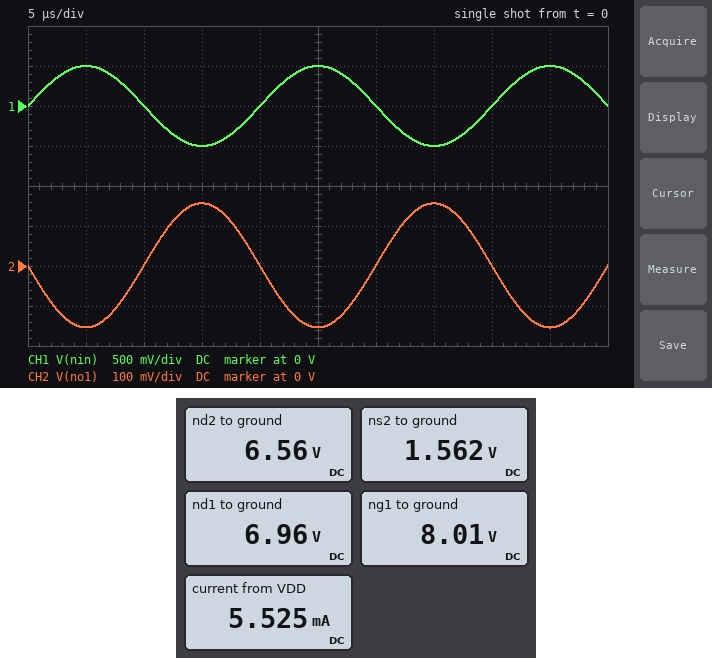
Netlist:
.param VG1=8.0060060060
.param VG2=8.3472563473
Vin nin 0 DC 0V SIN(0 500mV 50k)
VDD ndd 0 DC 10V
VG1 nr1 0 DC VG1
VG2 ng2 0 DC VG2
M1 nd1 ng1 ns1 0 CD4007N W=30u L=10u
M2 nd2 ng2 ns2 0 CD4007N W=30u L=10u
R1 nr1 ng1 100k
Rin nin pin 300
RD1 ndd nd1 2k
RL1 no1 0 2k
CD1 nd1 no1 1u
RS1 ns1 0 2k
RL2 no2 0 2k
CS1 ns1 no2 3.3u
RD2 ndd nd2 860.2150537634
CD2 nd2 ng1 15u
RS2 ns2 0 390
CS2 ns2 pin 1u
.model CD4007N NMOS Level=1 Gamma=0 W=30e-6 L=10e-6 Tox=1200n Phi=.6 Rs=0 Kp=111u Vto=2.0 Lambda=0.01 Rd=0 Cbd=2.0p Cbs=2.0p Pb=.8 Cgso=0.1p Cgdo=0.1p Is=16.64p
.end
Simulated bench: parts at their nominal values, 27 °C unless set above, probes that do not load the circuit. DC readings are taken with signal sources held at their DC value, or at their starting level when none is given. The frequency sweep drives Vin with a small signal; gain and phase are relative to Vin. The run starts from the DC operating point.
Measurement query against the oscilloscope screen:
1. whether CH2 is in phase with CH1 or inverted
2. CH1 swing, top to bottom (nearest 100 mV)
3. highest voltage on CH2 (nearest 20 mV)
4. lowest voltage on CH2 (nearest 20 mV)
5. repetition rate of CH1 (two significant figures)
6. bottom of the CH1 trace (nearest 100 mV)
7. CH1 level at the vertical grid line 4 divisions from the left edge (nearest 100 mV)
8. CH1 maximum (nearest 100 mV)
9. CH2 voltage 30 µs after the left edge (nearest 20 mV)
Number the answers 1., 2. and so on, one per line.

1. inverted
2. 1.0 V
3. 160 mV
4. -160 mV
5. 50 kHz
6. -500 mV
7. 0 V
8. 500 mV
9. 0 V
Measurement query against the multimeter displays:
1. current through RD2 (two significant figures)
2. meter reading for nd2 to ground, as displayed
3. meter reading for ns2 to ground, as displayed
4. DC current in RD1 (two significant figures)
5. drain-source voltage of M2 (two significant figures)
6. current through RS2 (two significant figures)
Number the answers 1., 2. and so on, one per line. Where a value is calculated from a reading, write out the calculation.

1. (10 V - 6.56 V) / 860.2 Ω = 4.0 mA
2. 6.56 V
3. 1.562 V
4. (10 V - 6.96 V) / 2 kΩ = 1.5 mA
5. 6.56 V - 1.562 V = 5.0 V
6. (1.562 V) / 390 Ω = 4.0 mA
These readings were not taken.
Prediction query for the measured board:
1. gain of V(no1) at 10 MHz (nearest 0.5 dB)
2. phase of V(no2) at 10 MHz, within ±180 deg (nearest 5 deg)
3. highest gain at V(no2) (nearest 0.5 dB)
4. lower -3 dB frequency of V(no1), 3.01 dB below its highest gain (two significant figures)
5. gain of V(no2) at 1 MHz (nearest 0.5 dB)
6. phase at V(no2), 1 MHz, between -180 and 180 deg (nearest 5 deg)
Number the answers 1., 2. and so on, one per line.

1. -10.0 dB
2. -5 deg
3. -10.0 dB
4. 300 Hz
5. -10.0 dB
6. 0 deg
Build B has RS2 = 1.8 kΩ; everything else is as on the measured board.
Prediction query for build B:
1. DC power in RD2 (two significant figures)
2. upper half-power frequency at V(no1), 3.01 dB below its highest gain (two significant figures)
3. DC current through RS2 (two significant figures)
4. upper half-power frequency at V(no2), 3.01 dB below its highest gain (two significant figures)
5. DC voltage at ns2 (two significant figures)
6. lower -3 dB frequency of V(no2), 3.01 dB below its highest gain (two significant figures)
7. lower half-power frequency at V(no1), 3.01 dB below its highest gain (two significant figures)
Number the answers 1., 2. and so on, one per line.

1. 2.7 mW
2. 280 MHz
3. 1.8 mA
4. 210 MHz
5. 3.2 V
6. 180 Hz
7. 190 Hz
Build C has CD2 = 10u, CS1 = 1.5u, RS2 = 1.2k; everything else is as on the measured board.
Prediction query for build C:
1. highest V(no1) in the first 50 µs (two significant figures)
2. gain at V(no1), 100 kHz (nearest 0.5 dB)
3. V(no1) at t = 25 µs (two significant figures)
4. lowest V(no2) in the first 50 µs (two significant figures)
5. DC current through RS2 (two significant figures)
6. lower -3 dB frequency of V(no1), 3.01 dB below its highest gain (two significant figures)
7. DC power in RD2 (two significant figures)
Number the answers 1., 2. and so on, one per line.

1. 170 mV
2. -9.5 dB
3. -160 mV
4. -170 mV
5. 2.3 mA
6. 220 Hz
7. 4.5 mW
